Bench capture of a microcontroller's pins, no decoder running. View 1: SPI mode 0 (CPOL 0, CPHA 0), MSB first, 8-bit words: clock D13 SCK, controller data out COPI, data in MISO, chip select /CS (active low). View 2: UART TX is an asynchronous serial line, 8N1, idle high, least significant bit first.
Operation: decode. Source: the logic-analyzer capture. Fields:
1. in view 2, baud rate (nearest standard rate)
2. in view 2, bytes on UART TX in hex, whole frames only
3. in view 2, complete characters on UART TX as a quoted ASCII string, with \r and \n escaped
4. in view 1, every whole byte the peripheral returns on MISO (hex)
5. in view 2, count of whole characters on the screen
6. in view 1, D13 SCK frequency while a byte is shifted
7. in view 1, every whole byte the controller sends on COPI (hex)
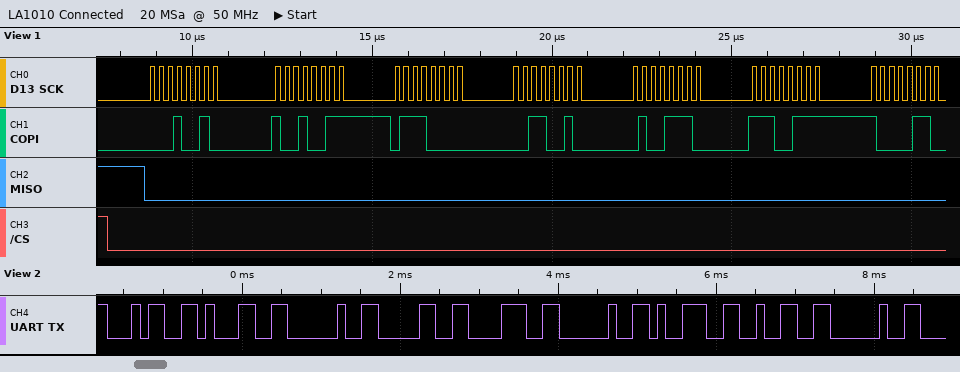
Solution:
9600 baud
34 31 20 30 38 20 39 32 20
"41 08 92 "
00 00 00 00 00 00 00
9
4 MHz
12 93 70 32 4E E7 86
